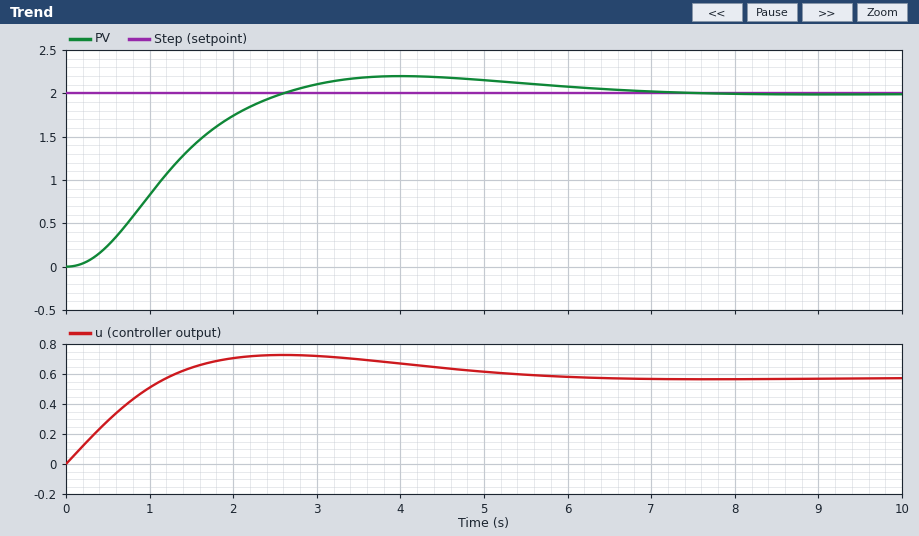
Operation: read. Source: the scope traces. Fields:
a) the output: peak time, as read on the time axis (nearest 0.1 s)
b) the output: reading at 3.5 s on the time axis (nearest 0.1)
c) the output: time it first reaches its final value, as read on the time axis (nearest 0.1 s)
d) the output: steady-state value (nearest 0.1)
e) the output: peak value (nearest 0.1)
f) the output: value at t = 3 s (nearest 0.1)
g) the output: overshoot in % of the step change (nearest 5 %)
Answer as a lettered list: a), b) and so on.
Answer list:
a) 4.0 s
b) 2.2
c) 2.6 s
d) 2.0
e) 2.2
f) 2.1
g) 10 %
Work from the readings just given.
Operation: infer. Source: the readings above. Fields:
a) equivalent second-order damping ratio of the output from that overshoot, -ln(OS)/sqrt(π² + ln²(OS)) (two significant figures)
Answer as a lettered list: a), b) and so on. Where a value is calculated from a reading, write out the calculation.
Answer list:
a) ln(0.1) = -2.303; 2.303 / sqrt(9.870 + 5.302) = 0.59
